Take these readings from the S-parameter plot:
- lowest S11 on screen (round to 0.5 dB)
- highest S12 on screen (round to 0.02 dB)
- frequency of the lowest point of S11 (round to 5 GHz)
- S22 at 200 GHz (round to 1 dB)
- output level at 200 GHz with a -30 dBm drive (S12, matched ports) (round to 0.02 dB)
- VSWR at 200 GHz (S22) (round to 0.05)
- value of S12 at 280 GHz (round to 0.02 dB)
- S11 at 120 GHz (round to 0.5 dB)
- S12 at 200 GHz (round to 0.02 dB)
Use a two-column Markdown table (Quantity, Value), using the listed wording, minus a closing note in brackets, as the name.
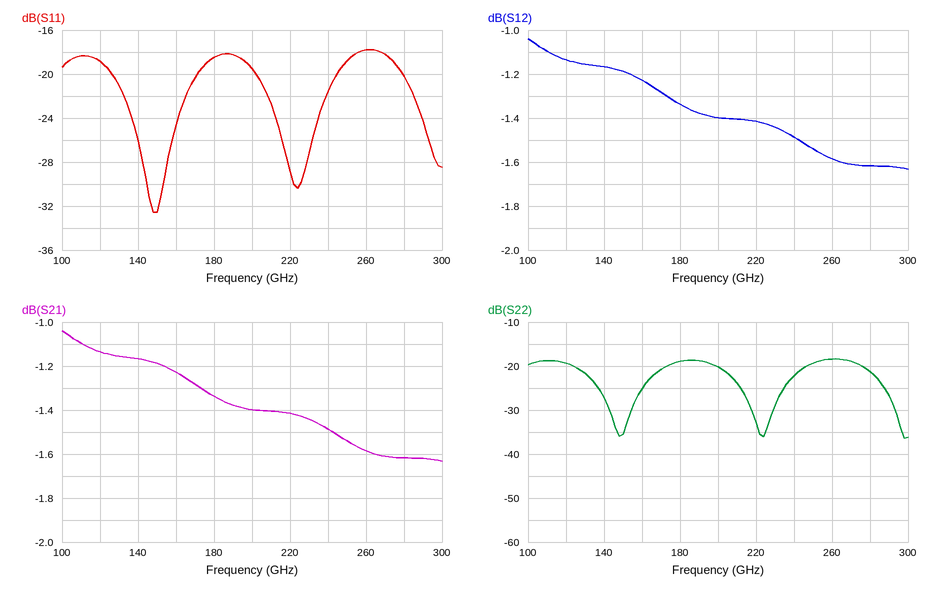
| Quantity | Value |
|---|---|
| lowest S11 on screen | -32.5 dB |
| highest S12 on screen | -1.04 dB |
| frequency of the lowest point of S11 | 150 GHz |
| S22 at 200 GHz | -20 dB |
| output level at 200 GHz with a -30 dBm drive (S12, matched ports) | -31.40 dBm |
| VSWR at 200 GHz (S22) | 1.20 |
| value of S12 at 280 GHz | -1.62 dB |
| S11 at 120 GHz | -19.0 dB |
| S12 at 200 GHz | -1.40 dB |
